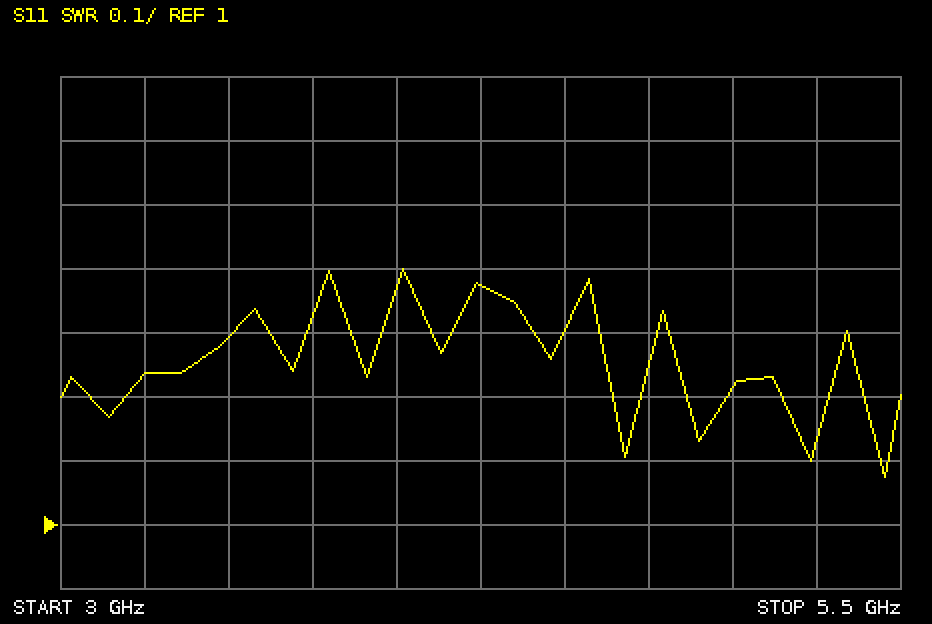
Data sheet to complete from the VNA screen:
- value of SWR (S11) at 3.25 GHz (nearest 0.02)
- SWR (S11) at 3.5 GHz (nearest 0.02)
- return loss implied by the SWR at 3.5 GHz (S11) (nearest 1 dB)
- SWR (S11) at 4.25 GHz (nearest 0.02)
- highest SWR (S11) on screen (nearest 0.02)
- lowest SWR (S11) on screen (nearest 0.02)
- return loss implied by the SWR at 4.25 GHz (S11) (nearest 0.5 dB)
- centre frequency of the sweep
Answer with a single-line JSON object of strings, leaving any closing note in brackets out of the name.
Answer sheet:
{"value of SWR (S11) at 3.25 GHz": "1.24", "SWR (S11) at 3.5 GHz": "1.30", "return loss implied by the SWR at 3.5 GHz (S11)": "18 dB", "SWR (S11) at 4.25 GHz": "1.38", "highest SWR (S11) on screen": "1.40", "lowest SWR (S11) on screen": "1.08", "return loss implied by the SWR at 4.25 GHz (S11)": "16.0 dB", "centre frequency of the sweep": "4.25 GHz"}
